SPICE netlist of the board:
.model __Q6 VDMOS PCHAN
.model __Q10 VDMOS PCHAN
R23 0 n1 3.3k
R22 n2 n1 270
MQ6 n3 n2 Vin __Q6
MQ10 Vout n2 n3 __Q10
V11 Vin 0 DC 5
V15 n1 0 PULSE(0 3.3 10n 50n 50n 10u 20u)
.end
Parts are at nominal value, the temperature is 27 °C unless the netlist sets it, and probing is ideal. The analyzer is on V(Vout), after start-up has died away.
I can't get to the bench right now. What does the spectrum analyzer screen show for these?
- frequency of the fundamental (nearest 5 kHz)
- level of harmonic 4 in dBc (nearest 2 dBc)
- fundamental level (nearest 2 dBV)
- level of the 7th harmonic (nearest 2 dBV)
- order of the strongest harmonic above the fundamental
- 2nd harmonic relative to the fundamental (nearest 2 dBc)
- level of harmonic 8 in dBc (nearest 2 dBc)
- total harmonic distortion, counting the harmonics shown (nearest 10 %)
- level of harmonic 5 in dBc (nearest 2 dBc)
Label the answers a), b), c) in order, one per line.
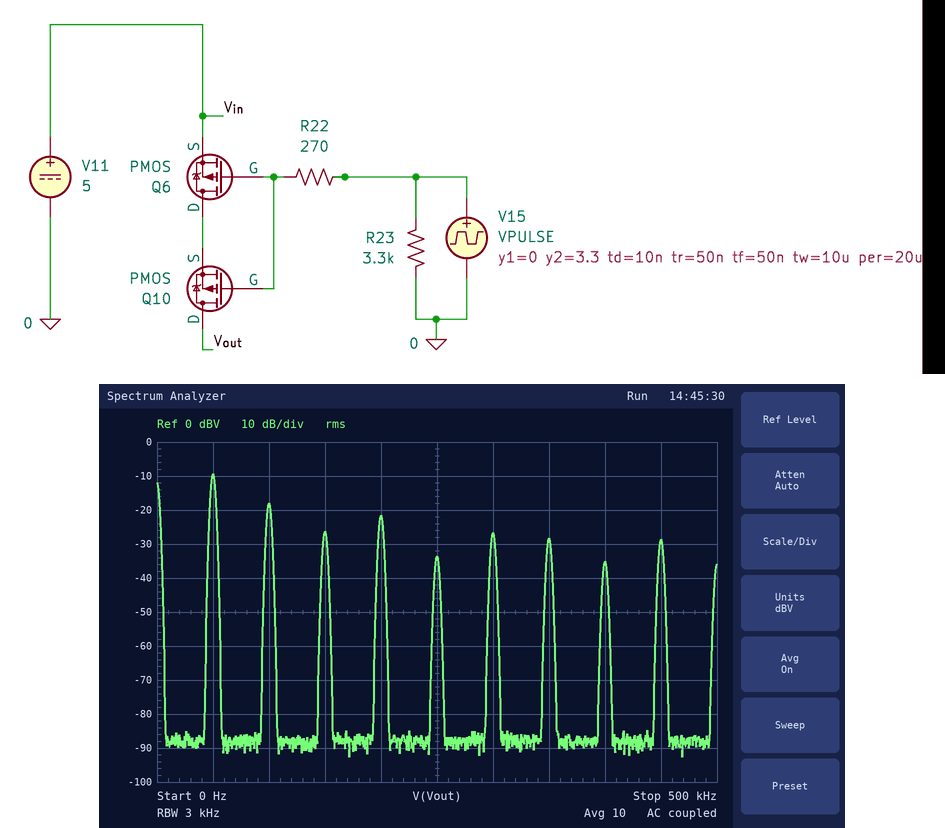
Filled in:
a) 50 kHz
b) -12 dBc
c) -10 dBV
d) -28 dBV
e) 2
f) -8 dBc
g) -26 dBc
h) 50 %
i) -24 dBc
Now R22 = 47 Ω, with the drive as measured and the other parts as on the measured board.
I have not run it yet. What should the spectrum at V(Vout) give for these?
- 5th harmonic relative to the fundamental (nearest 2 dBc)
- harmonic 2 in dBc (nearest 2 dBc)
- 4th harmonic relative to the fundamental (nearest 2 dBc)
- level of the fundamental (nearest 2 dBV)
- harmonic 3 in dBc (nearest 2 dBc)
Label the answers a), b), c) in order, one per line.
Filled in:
a) -14 dBc
b) -24 dBc
c) -24 dBc
d) -8 dBV
e) -10 dBc
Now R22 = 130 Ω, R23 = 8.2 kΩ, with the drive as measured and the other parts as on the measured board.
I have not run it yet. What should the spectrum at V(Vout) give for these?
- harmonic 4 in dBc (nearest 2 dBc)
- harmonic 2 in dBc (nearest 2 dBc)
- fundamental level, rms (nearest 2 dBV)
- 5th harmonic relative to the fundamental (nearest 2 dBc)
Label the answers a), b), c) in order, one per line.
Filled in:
a) -16 dBc
b) -14 dBc
c) -8 dBV
d) -18 dBc
